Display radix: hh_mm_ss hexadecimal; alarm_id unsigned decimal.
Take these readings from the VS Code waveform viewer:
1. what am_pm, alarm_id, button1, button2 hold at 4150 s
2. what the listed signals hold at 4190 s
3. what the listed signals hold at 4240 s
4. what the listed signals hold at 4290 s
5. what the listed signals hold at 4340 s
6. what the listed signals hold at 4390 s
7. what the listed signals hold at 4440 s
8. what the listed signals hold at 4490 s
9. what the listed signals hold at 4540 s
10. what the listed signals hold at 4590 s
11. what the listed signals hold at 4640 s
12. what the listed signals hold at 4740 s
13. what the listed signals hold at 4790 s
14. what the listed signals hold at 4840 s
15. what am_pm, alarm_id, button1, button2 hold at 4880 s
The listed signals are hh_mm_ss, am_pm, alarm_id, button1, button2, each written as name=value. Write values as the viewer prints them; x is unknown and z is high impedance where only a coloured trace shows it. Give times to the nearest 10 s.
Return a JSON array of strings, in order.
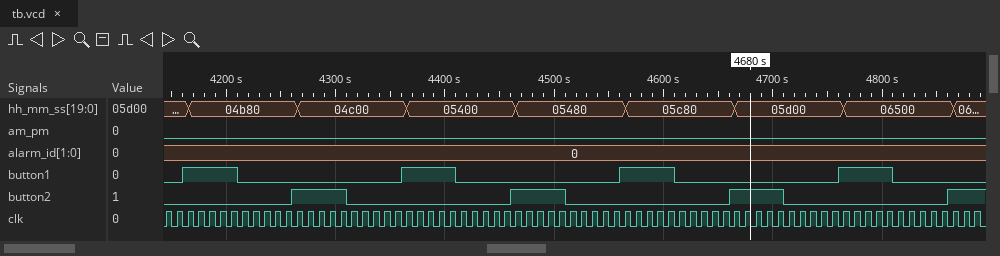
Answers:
["am_pm=0, alarm_id=0, button1=0, button2=0", "hh_mm_ss=04b80, am_pm=0, alarm_id=0, button1=1, button2=0", "hh_mm_ss=04b80, am_pm=0, alarm_id=0, button1=0, button2=0", "hh_mm_ss=04c00, am_pm=0, alarm_id=0, button1=0, button2=1", "hh_mm_ss=04c00, am_pm=0, alarm_id=0, button1=0, button2=0", "hh_mm_ss=05400, am_pm=0, alarm_id=0, button1=1, button2=0", "hh_mm_ss=05400, am_pm=0, alarm_id=0, button1=0, button2=0", "hh_mm_ss=05480, am_pm=0, alarm_id=0, button1=0, button2=1", "hh_mm_ss=05480, am_pm=0, alarm_id=0, button1=0, button2=0", "hh_mm_ss=05c80, am_pm=0, alarm_id=0, button1=1, button2=0", "hh_mm_ss=05c80, am_pm=0, alarm_id=0, button1=0, button2=0", "hh_mm_ss=05d00, am_pm=0, alarm_id=0, button1=0, button2=0", "hh_mm_ss=06500, am_pm=0, alarm_id=0, button1=1, button2=0", "hh_mm_ss=06500, am_pm=0, alarm_id=0, button1=0, button2=0", "am_pm=0, alarm_id=0, button1=0, button2=1"]
